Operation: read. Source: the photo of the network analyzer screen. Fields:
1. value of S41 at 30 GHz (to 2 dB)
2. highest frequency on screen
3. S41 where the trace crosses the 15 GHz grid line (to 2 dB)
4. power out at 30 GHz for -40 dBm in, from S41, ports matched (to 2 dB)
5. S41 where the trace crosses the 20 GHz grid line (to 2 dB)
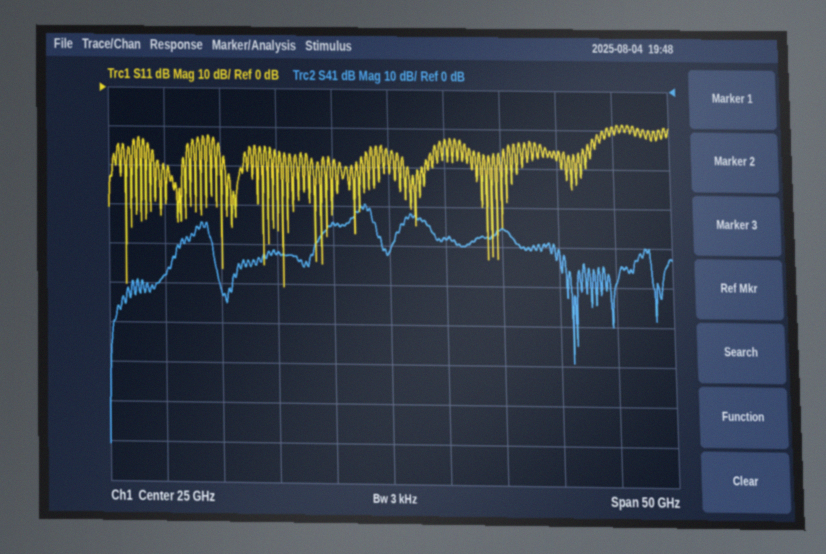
-38 dB
50 GHz
-42 dB
-78 dBm
-34 dB
